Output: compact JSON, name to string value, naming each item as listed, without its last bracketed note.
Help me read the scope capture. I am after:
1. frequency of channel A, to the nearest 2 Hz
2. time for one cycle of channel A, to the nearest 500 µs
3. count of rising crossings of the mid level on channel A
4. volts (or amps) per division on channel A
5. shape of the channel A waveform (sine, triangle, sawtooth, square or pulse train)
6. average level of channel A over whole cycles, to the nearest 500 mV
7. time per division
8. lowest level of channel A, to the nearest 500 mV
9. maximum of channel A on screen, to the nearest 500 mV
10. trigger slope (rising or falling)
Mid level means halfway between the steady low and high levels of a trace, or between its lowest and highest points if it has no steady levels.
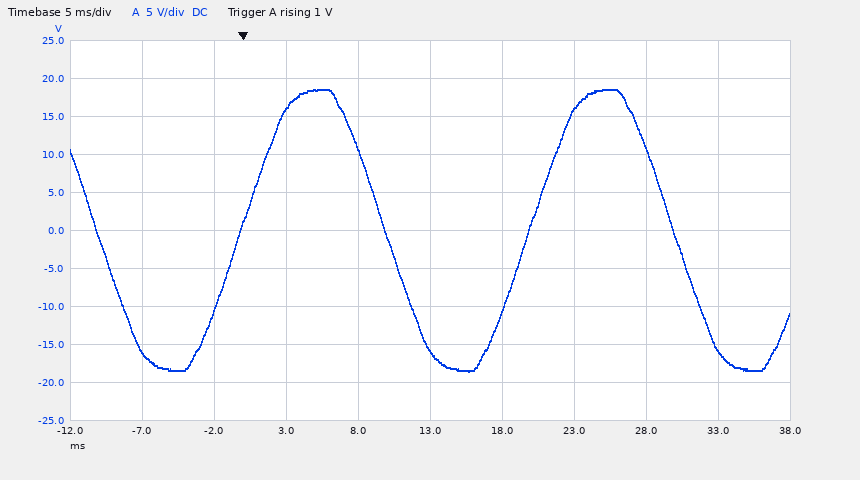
{"frequency of channel A, to the nearest 2 Hz": "50 Hz", "time for one cycle of channel A, to the nearest 500 µs": "20.0 ms", "count of rising crossings of the mid level on channel A": "2", "volts (or amps) per division on channel A": "5 V", "shape of the channel A waveform": "sine", "average level of channel A over whole cycles, to the nearest 500 mV": "0.0 V", "time per division": "5 ms", "lowest level of channel A, to the nearest 500 mV": "-18.5 V", "maximum of channel A on screen, to the nearest 500 mV": "18.5 V", "trigger slope": "rising"}
